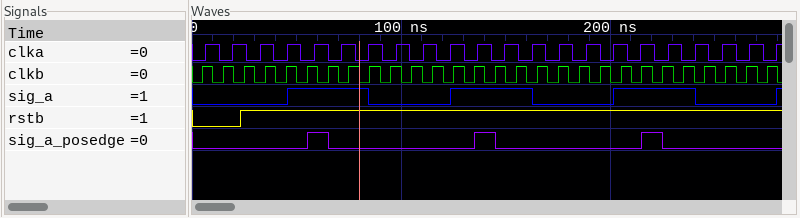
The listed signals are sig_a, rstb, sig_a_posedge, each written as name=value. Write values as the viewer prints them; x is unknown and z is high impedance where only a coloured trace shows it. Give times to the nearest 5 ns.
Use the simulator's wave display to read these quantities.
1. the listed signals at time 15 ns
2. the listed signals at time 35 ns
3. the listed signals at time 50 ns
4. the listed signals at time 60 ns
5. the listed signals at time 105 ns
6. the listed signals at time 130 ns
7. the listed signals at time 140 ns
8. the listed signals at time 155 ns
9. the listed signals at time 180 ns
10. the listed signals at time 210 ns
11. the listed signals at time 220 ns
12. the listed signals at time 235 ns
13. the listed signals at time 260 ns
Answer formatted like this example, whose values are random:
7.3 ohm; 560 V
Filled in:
sig_a=0, rstb=0, sig_a_posedge=0; sig_a=0, rstb=1, sig_a_posedge=0; sig_a=1, rstb=1, sig_a_posedge=0; sig_a=1, rstb=1, sig_a_posedge=1; sig_a=0, rstb=1, sig_a_posedge=0; sig_a=1, rstb=1, sig_a_posedge=0; sig_a=1, rstb=1, sig_a_posedge=1; sig_a=1, rstb=1, sig_a_posedge=0; sig_a=0, rstb=1, sig_a_posedge=0; sig_a=1, rstb=1, sig_a_posedge=0; sig_a=1, rstb=1, sig_a_posedge=1; sig_a=1, rstb=1, sig_a_posedge=0; sig_a=0, rstb=1, sig_a_posedge=0
